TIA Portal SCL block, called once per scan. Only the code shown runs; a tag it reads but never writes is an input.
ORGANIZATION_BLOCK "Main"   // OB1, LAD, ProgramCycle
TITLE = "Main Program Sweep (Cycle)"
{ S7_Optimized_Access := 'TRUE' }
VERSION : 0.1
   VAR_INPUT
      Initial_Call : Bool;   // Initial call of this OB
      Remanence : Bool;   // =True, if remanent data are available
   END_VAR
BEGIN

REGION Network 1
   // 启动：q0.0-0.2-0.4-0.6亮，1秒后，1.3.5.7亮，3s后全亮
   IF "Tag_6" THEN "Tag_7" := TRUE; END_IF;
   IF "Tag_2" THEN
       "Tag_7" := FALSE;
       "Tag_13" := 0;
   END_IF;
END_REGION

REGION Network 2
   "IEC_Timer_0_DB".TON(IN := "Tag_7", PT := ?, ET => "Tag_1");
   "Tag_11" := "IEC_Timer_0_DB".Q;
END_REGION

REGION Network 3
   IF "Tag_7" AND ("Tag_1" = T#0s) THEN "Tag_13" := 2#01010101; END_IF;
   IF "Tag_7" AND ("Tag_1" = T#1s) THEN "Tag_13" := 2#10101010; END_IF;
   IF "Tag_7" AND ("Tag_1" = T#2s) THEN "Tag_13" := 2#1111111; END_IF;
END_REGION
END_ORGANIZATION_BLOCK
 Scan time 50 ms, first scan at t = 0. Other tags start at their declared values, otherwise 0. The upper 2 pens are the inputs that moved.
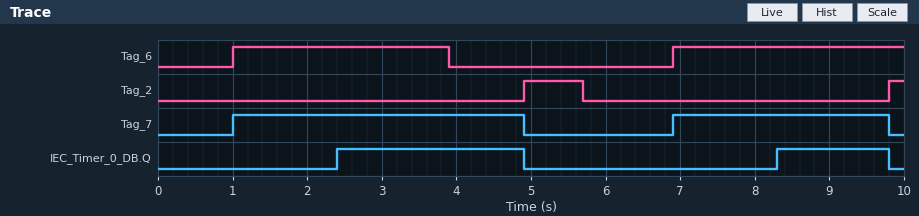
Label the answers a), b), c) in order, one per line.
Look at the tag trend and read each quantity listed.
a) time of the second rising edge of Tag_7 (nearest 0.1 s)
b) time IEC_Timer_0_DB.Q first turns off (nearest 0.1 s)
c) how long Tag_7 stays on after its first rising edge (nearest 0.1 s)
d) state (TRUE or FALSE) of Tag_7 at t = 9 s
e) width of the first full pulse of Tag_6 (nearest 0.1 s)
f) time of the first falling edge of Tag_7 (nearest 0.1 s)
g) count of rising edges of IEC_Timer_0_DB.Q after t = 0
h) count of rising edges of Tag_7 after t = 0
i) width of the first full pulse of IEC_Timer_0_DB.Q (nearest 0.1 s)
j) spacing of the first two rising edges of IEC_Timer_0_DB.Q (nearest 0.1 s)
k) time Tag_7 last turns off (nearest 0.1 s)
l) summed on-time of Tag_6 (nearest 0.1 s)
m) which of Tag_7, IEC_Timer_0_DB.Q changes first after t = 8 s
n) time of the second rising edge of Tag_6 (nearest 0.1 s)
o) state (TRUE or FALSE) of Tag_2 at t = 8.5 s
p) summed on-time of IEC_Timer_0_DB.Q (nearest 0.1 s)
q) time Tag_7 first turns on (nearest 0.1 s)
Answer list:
a) 6.9 s
b) 4.9 s
c) 3.9 s
d) TRUE
e) 2.9 s
f) 4.9 s
g) 2
h) 2
i) 2.5 s
j) 5.9 s
k) 9.8 s
l) 6.0 s
m) IEC_Timer_0_DB.Q
n) 6.9 s
o) FALSE
p) 4.0 s
q) 1.0 s
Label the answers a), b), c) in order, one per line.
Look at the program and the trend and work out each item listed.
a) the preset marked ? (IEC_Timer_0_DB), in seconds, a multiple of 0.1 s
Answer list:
a) 1.4 s
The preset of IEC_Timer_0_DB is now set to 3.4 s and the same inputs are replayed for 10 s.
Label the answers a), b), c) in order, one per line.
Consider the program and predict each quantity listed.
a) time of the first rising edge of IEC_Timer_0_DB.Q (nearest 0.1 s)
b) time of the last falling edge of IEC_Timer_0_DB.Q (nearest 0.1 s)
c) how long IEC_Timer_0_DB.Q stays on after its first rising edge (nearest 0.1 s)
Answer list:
a) 4.4 s
b) 4.9 s
c) 0.5 s
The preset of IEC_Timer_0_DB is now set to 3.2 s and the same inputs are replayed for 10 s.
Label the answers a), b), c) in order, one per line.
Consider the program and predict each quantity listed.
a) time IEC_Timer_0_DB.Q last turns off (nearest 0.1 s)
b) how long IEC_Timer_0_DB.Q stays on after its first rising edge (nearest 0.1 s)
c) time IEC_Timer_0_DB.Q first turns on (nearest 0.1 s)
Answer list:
a) 4.9 s
b) 0.7 s
c) 4.2 s
